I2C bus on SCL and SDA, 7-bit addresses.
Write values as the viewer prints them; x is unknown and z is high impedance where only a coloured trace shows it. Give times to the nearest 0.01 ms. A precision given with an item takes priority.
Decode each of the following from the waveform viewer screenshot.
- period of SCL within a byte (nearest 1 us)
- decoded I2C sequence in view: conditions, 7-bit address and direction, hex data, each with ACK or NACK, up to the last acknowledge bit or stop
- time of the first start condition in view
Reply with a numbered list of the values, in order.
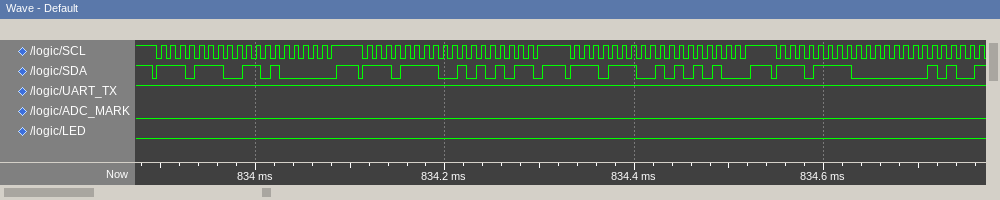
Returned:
1. 10 us
2. start, address 77 write ACK, D0 ACK, stop, start, address 77 read ACK, 55 NACK, stop, start, address 77 write ACK, AA ACK, stop, start, address 77 read ACK, 01 ACK
3. 833.89 ms
